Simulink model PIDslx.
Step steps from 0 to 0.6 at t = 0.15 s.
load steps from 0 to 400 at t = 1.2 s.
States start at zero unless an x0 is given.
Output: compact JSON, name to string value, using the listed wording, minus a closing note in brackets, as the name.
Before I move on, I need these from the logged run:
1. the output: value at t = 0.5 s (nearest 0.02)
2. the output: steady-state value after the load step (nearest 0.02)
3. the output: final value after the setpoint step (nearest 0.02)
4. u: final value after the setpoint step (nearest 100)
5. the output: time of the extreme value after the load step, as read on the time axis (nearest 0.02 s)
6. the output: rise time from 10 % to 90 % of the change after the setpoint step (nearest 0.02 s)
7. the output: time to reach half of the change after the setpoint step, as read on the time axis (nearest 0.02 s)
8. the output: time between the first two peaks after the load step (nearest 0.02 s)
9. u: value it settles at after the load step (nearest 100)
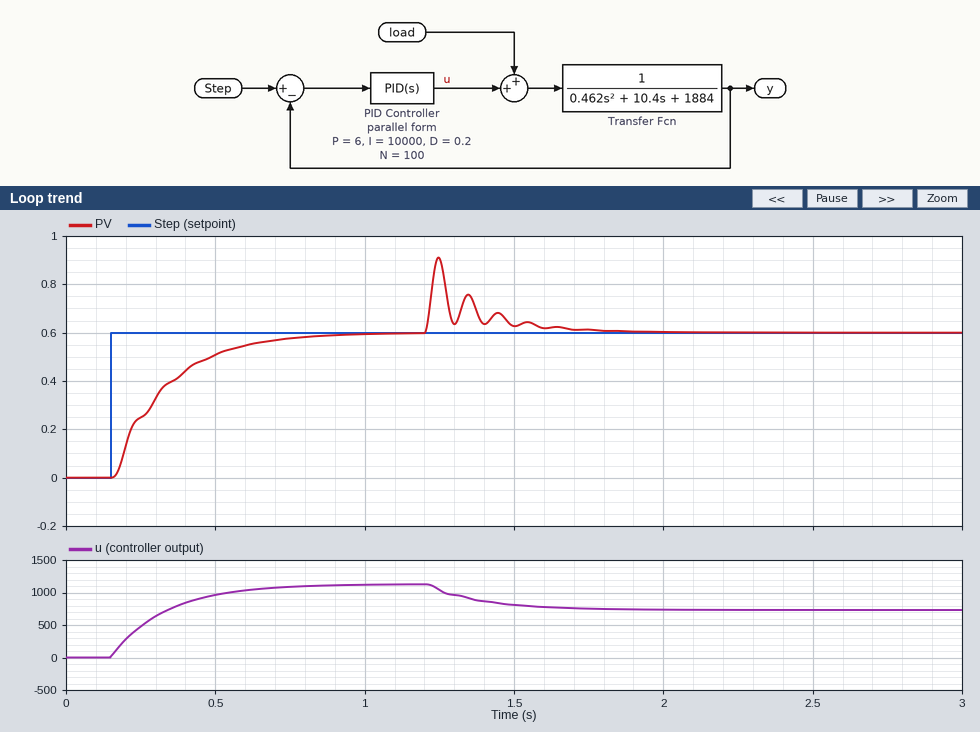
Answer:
{"the output: value at t = 0.5 s": "0.50", "the output: steady-state value after the load step": "0.60", "the output: final value after the setpoint step": "0.60", "u: final value after the setpoint step": "1100", "the output: time of the extreme value after the load step, as read on the time axis": "1.24 s", "the output: rise time from 10 % to 90 % of the change after the setpoint step": "0.40 s", "the output: time to reach half of the change after the setpoint step, as read on the time axis": "0.28 s", "the output: time between the first two peaks after the load step": "0.10 s", "u: value it settles at after the load step": "700"}
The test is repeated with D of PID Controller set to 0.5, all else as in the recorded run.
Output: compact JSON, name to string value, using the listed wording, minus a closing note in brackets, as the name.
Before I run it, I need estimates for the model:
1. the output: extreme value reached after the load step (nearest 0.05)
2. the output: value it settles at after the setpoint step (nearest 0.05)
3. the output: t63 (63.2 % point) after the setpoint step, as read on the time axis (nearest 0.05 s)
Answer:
{"the output: extreme value reached after the load step": "0.90", "the output: value it settles at after the setpoint step": "0.60", "the output: t63 (63.2 % point) after the setpoint step, as read on the time axis": "0.35 s"}
